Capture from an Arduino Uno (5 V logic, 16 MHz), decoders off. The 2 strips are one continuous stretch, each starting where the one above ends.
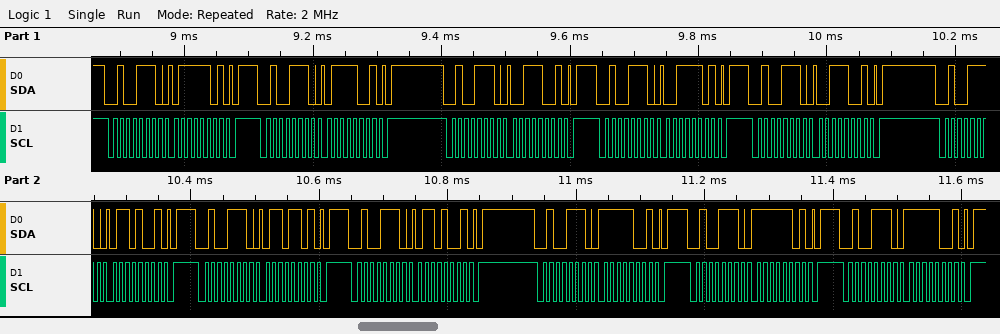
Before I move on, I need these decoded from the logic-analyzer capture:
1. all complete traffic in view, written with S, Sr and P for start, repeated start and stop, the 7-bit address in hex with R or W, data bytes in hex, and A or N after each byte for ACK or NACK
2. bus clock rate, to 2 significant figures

S 27W A 7D A P S 27W A 79 A P S 27W A 39 A P S 27W A 3D A P S 27W A 39 A P S 27W A 69 A P S 27W A 6D A P S 27W A 69 A P S 27W A F9 A P S 27W A FD A P S 27W A F9 A P
100 kHz
